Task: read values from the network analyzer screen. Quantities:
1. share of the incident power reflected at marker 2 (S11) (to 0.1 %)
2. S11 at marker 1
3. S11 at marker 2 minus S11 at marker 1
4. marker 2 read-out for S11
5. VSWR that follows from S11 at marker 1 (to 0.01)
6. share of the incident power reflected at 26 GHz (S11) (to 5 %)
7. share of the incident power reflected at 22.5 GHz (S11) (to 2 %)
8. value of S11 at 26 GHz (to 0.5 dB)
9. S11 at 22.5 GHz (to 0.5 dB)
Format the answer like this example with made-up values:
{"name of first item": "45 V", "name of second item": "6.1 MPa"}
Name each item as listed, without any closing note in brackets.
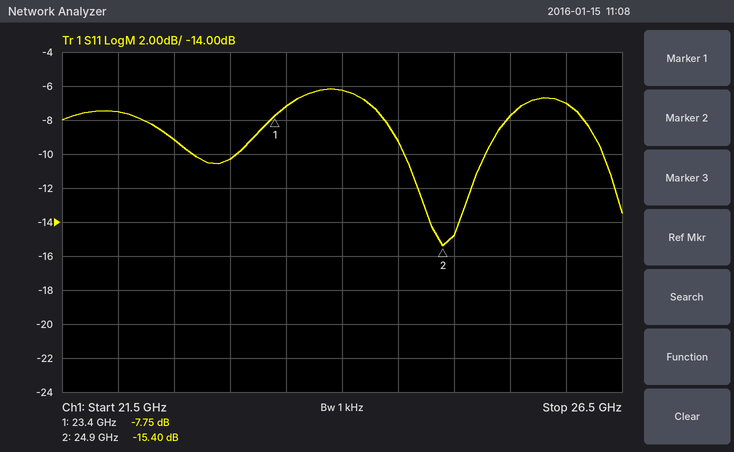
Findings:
{"share of the incident power reflected at marker 2 (S11)": "2.9 %", "S11 at marker 1": "-7.75 dB", "S11 at marker 2 minus S11 at marker 1": "-7.65 dB", "marker 2 read-out for S11": "-15.40 dB", "VSWR that follows from S11 at marker 1": "2.39", "share of the incident power reflected at 26 GHz (S11)": "20 %", "share of the incident power reflected at 22.5 GHz (S11)": "12 %", "value of S11 at 26 GHz": "-7.0 dB", "S11 at 22.5 GHz": "-9.0 dB"}
